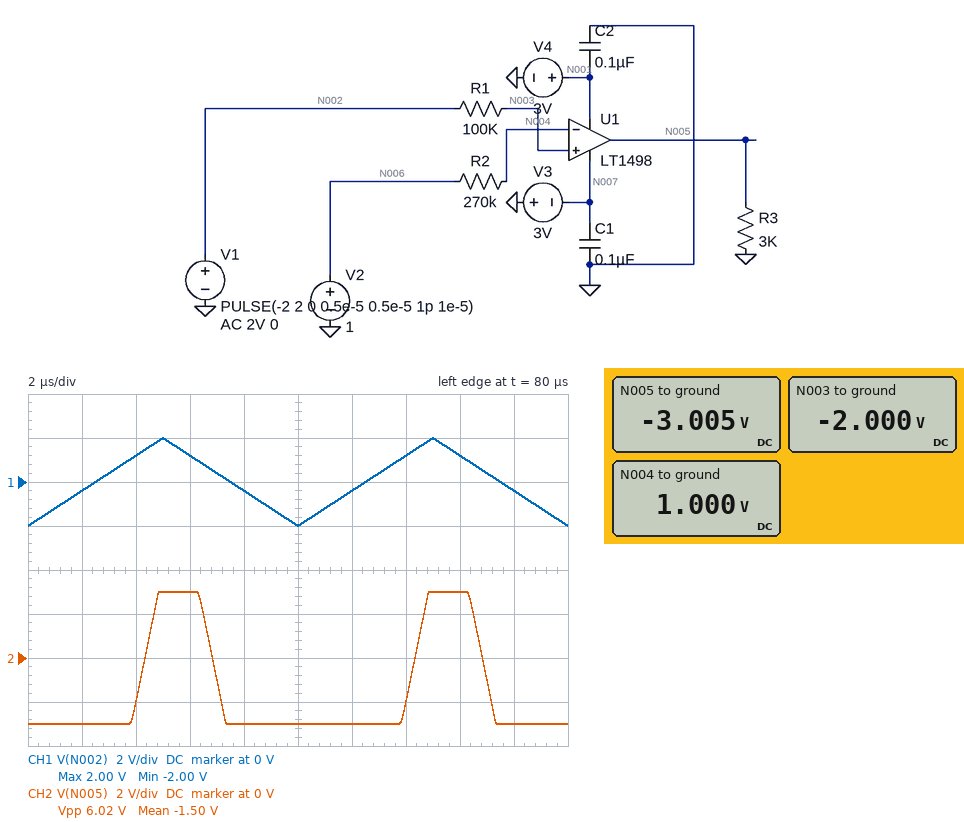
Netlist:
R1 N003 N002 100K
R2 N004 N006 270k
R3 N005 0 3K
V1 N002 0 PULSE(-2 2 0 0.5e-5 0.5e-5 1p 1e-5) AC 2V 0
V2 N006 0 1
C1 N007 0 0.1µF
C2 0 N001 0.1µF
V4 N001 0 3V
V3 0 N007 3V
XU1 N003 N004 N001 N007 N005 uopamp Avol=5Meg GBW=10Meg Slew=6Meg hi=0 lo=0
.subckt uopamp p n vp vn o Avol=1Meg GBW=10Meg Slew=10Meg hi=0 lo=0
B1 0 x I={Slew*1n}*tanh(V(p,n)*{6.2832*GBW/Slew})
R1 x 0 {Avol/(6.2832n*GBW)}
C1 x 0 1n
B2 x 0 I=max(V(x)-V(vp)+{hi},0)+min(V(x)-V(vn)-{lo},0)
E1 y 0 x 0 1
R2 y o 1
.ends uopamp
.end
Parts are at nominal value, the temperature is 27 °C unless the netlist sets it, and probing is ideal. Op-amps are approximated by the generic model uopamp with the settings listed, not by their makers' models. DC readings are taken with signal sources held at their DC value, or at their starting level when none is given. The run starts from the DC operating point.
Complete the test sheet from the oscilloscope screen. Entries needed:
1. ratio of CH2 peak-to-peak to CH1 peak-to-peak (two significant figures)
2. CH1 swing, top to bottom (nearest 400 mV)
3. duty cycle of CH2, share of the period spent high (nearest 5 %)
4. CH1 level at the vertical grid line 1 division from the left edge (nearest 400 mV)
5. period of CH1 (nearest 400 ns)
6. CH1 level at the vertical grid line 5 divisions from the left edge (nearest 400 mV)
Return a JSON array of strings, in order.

["1.5", "4.0 V", "25 %", "-400 mV", "10.0 µs", "-2.0 V"]
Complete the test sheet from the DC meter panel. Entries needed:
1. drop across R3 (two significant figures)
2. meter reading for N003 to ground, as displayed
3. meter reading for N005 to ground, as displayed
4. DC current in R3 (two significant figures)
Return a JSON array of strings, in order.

["3.0 V", "-2.000 V", "-3.005 V", "1.0 mA"]
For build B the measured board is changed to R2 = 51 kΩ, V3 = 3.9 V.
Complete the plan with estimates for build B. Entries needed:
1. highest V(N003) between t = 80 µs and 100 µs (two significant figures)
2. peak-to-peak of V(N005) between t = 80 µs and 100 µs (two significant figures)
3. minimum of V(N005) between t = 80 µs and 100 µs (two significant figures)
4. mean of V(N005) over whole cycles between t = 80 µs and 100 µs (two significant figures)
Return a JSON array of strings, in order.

["2.0 V", "6.9 V", "-3.9 V", "-2.2 V"]
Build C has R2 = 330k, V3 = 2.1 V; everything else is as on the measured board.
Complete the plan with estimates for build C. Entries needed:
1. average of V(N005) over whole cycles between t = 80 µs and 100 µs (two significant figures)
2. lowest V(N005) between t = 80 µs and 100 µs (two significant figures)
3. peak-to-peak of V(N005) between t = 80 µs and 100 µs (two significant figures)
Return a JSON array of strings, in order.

["-830 mV", "-2.1 V", "5.1 V"]
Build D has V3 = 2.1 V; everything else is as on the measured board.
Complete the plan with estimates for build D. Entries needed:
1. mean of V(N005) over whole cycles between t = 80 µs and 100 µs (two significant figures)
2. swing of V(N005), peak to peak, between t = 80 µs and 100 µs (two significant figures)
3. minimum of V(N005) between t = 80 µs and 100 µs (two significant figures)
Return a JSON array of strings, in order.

["-830 mV", "5.1 V", "-2.1 V"]
